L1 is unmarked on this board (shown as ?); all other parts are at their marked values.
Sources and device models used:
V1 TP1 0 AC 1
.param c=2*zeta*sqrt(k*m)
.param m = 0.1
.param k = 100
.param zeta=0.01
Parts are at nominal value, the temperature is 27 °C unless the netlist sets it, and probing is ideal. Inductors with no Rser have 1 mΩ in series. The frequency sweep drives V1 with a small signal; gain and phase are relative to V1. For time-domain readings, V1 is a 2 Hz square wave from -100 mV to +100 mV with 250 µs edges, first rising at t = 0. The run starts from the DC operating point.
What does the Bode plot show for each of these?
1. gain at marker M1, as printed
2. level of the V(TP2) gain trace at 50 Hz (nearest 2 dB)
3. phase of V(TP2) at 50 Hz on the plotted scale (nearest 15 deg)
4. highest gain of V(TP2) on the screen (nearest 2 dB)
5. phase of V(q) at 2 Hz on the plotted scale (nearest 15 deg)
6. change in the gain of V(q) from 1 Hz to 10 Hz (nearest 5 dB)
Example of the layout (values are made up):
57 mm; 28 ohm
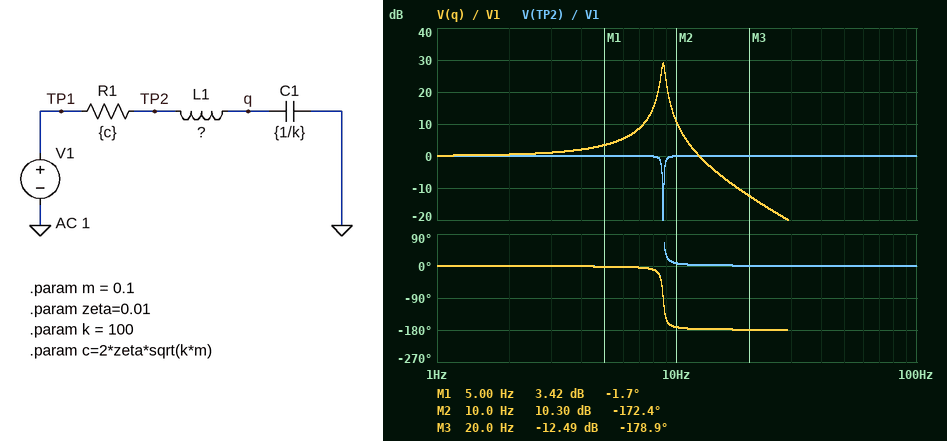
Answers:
3.42 dB; 0 dB; 0 deg; 0 dB; 0 deg; 10 dB
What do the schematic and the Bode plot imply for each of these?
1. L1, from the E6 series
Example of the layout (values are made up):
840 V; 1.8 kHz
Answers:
33 mH
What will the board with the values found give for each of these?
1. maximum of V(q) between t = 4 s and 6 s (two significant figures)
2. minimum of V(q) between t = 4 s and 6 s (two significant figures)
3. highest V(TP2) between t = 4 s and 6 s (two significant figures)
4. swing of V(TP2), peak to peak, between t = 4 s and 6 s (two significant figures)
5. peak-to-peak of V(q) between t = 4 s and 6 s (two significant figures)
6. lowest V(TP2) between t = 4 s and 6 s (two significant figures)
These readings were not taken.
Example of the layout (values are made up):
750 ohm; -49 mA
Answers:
230 mV; -230 mV; 100 mV; 210 mV; 450 mV; -100 mV
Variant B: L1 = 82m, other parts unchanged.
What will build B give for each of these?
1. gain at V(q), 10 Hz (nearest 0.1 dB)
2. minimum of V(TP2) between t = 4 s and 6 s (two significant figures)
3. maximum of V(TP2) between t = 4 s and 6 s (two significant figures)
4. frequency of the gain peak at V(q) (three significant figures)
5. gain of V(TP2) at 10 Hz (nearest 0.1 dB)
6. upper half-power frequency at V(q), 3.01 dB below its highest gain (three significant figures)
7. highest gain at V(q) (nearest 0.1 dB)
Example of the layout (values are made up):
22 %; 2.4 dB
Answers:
-7.0 dB; -110 mV; 110 mV; 5.56 Hz; 0 dB; 5.62 Hz; 33.0 dB
